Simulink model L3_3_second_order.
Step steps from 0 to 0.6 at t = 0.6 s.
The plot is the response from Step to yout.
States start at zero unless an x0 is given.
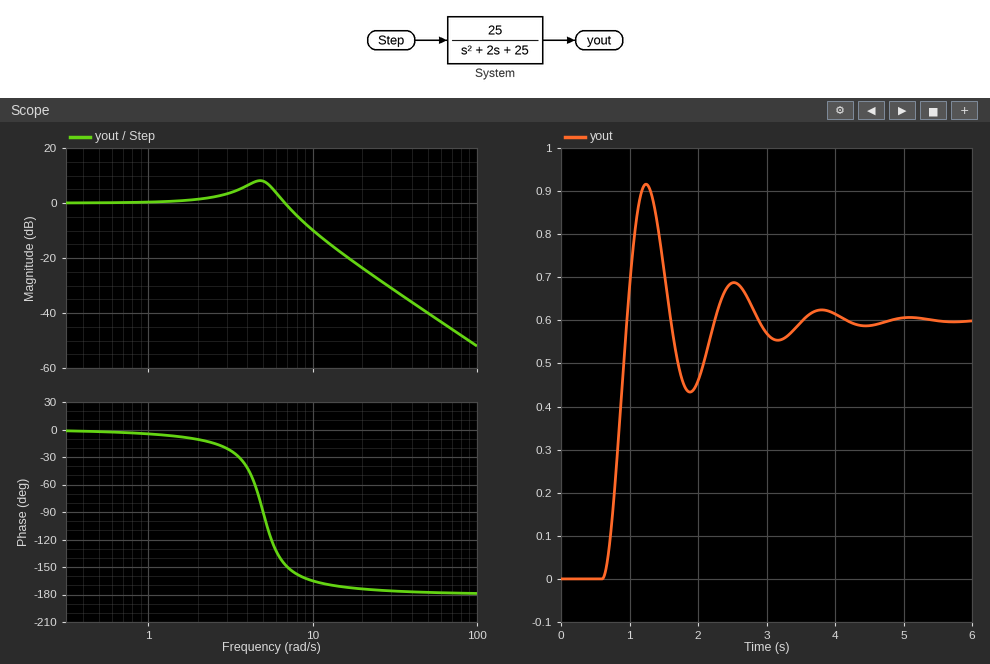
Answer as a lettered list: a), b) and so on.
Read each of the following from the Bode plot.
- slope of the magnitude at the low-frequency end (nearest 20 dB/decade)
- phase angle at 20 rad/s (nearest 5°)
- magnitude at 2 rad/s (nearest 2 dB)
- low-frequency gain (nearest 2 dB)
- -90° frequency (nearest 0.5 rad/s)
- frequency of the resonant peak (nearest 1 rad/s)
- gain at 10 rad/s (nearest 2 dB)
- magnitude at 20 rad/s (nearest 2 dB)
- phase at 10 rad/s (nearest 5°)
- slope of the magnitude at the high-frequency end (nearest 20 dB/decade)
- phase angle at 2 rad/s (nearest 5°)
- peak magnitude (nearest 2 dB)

a) 0 dB/decade
b) -175°
c) 2 dB
d) 0 dB
e) 5.0 rad/s
f) 5 rad/s
g) -10 dB
h) -24 dB
i) -165°
j) -40 dB/decade
k) -10°
l) 8 dB
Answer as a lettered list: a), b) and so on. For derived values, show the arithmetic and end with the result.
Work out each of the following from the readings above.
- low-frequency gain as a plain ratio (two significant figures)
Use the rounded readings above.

a) 10^(0 / 20) = 1.0
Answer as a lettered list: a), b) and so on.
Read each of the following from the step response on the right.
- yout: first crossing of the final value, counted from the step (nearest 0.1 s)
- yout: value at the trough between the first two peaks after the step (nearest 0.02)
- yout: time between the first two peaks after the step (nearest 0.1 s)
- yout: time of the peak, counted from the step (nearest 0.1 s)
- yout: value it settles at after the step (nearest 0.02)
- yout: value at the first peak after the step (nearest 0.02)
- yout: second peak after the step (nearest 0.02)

a) 0.4 s
b) 0.44
c) 1.3 s
d) 0.6 s
e) 0.60
f) 0.92
g) 0.68
